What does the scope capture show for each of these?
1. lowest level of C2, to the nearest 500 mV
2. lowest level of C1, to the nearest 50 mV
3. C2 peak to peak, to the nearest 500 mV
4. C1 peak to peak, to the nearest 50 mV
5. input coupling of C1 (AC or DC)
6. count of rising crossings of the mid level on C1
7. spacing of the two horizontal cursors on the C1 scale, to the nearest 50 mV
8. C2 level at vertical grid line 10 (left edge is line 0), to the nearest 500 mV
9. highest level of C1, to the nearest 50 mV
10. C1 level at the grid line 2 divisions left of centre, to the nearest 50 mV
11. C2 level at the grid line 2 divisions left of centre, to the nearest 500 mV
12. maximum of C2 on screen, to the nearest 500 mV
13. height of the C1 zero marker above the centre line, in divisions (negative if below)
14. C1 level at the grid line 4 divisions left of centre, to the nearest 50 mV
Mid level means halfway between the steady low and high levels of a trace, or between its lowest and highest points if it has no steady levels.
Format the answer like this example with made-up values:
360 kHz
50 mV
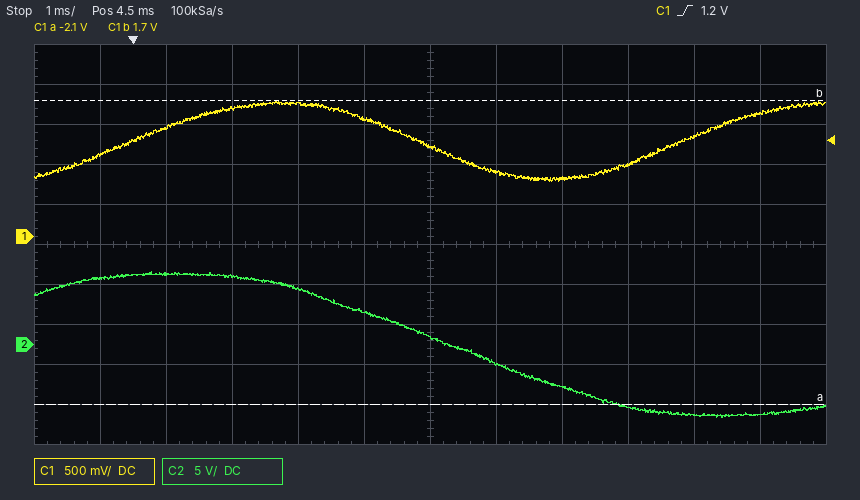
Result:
-9.0 V
700 mV
18.0 V
1.00 V
DC
2
3.80 V
-9.0 V
1.70 V
1.65 V
7.0 V
9.0 V
+0.2 div
1.35 V
